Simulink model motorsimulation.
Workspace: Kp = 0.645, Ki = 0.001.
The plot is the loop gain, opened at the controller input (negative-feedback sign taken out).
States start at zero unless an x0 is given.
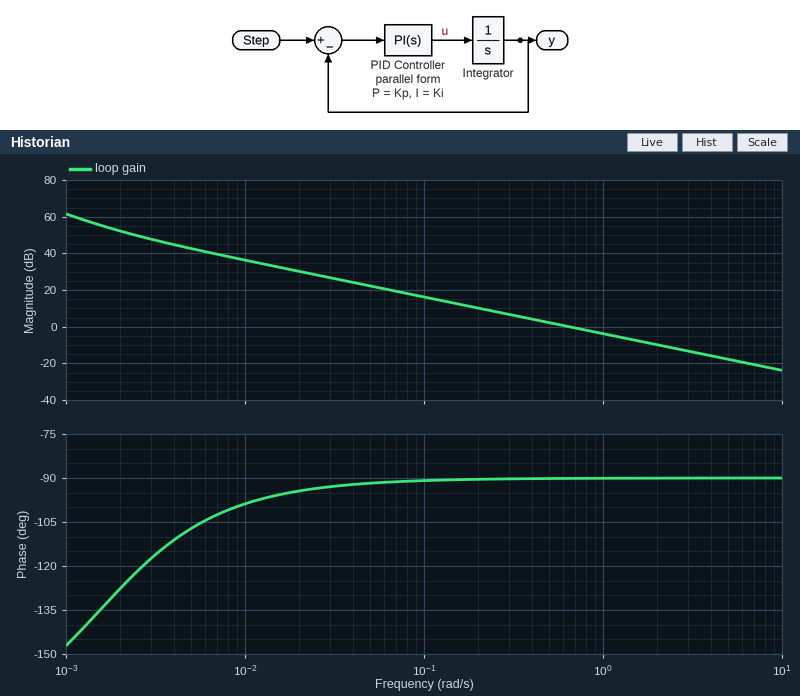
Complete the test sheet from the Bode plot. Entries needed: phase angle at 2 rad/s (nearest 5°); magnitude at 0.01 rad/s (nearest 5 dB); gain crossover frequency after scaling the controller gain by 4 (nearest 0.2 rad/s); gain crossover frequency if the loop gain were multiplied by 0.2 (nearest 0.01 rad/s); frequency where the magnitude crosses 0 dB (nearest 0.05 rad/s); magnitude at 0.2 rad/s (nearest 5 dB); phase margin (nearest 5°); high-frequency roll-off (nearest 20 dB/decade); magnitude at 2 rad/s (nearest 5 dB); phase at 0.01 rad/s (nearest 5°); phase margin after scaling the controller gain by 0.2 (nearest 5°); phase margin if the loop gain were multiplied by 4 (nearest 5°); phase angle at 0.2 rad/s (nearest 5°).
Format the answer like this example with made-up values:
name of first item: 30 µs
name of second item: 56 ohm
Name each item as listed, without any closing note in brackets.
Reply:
phase angle at 2 rad/s: -90°
magnitude at 0.01 rad/s: 35 dB
gain crossover frequency after scaling the controller gain by 4: 2.6 rad/s
gain crossover frequency if the loop gain were multiplied by 0.2: 0.13 rad/s
frequency where the magnitude crosses 0 dB: 0.65 rad/s
magnitude at 0.2 rad/s: 10 dB
phase margin: 90°
high-frequency roll-off: -20 dB/decade
magnitude at 2 rad/s: -10 dB
phase at 0.01 rad/s: -100°
phase margin after scaling the controller gain by 0.2: 90°
phase margin if the loop gain were multiplied by 4: 90°
phase angle at 0.2 rad/s: -90°
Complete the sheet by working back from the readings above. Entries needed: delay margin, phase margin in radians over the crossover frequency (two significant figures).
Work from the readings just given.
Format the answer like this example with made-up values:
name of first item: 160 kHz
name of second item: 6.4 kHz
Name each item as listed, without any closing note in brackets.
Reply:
delay margin, phase margin in radians over the crossover frequency: 2.4 s
